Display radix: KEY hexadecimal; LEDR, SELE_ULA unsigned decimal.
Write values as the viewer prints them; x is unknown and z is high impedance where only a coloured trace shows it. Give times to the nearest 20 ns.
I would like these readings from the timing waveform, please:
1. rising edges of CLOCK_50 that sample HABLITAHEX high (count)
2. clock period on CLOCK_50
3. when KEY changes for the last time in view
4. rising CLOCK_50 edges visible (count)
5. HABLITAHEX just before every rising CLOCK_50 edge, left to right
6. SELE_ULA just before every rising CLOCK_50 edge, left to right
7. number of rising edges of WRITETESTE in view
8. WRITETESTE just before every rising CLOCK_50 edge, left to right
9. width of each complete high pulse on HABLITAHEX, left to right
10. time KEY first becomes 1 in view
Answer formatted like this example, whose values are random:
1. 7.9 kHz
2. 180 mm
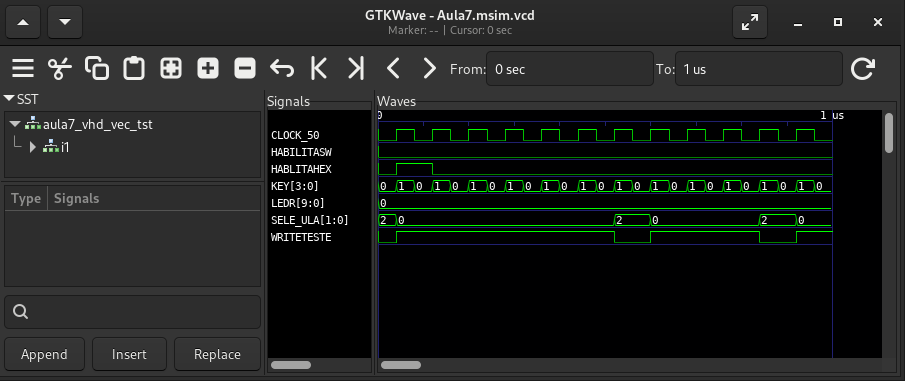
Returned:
1. 1
2. 80 ns
3. 960 ns
4. 12
5. 0 1 0 0 0 0 0 0 0 0 0 0
6. 2, 0, 0, 0, 0, 0, 0, 2, 0, 0, 0, 2
7. 3
8. 0 1 1 1 1 1 1 0 1 1 1 0
9. 80 ns
10. 40 ns
